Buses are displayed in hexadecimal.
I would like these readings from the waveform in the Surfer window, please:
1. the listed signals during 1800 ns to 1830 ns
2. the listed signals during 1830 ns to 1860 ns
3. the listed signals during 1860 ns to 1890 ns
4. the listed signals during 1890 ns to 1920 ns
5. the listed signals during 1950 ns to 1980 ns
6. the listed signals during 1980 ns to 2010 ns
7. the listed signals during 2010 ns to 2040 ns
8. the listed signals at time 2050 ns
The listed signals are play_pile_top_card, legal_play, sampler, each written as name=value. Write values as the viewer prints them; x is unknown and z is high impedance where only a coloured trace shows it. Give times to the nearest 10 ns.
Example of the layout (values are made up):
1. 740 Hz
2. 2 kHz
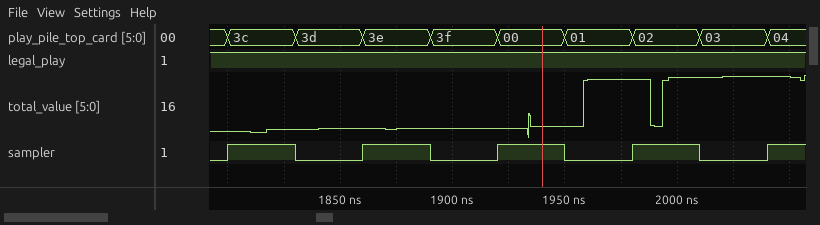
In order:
1. play_pile_top_card=3c, legal_play=1, sampler=1
2. play_pile_top_card=3d, legal_play=1, sampler=0
3. play_pile_top_card=3e, legal_play=1, sampler=1
4. play_pile_top_card=3f, legal_play=1, sampler=0
5. play_pile_top_card=01, legal_play=1, sampler=0
6. play_pile_top_card=02, legal_play=1, sampler=1
7. play_pile_top_card=03, legal_play=1, sampler=0
8. play_pile_top_card=04, legal_play=1, sampler=1
